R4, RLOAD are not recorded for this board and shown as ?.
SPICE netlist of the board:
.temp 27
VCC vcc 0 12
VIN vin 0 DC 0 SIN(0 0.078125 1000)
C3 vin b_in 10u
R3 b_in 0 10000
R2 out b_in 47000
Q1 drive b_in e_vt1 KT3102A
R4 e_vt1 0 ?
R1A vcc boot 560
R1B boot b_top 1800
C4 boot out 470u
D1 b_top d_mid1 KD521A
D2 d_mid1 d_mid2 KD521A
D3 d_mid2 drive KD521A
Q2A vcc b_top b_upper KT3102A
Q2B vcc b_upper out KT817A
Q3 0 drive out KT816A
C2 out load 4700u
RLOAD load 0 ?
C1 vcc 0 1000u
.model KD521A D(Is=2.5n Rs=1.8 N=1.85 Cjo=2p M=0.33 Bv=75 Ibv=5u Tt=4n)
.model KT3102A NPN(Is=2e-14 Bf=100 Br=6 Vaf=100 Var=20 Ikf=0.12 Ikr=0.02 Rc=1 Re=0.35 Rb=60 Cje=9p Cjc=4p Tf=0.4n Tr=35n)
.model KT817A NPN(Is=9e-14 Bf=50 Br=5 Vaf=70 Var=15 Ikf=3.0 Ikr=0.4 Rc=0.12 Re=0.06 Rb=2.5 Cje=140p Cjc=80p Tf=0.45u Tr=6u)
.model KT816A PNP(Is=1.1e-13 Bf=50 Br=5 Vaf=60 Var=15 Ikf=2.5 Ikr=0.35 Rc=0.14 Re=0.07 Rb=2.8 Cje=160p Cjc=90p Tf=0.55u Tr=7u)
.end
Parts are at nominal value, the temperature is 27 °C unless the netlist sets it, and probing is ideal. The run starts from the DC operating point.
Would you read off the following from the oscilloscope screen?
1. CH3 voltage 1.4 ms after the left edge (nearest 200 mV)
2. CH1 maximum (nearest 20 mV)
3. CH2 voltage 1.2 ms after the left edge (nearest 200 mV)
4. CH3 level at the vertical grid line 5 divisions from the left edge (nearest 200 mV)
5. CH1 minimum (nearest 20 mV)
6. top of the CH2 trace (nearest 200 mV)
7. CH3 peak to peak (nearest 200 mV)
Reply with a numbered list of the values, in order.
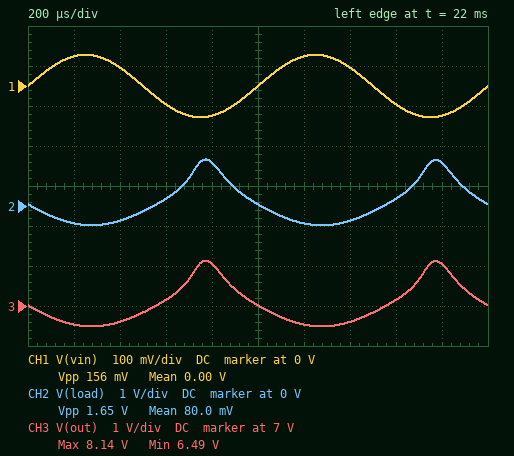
1. 6.6 V
2. 80 mV
3. -400 mV
4. 7.0 V
5. -80 mV
6. 1.2 V
7. 1.6 V
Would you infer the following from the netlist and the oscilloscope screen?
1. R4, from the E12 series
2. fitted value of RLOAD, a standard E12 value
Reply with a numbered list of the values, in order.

1. 220 Ω
2. 22 Ω
